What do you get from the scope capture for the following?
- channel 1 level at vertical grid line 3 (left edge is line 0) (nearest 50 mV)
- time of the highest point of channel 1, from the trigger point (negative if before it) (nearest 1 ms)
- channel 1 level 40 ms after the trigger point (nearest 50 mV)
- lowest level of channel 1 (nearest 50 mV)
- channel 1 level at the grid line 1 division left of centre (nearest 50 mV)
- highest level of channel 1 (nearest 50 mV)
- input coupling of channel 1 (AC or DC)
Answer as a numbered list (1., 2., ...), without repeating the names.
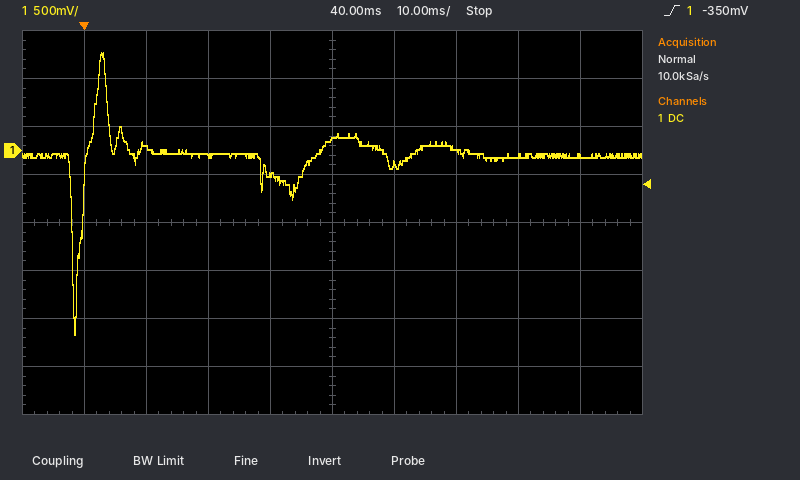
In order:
1. -50 mV
2. +3 ms
3. 100 mV
4. -1.90 V
5. -250 mV
6. 1.00 V
7. DC
